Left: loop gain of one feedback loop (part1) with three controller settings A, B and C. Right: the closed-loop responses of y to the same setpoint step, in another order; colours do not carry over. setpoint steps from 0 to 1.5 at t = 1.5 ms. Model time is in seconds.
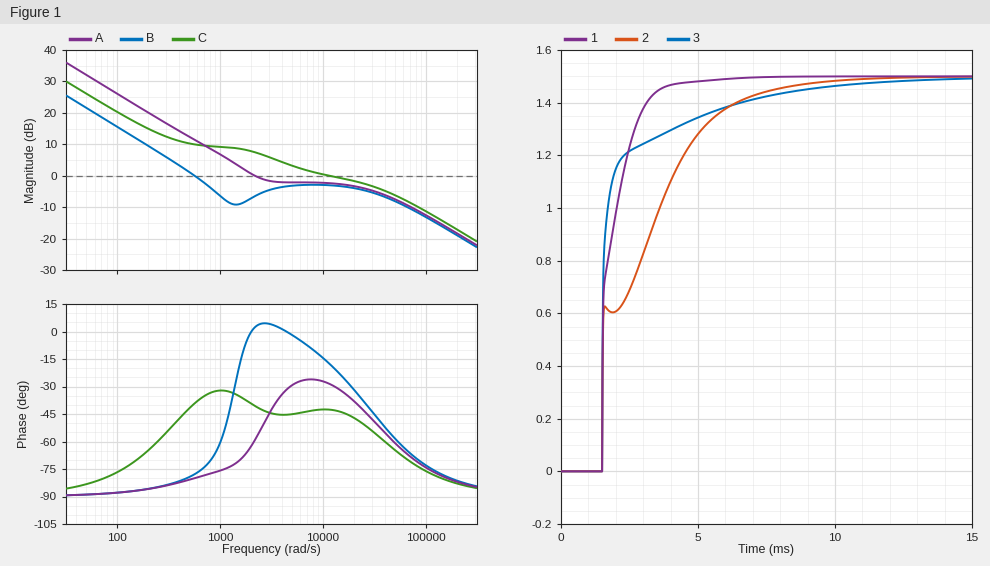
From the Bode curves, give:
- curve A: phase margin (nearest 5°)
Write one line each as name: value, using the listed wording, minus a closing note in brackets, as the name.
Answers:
curve A: phase margin: 120°
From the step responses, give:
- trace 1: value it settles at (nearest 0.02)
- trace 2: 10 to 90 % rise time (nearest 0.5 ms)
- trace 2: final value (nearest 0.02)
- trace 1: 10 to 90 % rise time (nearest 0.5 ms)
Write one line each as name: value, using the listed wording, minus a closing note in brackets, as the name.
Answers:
trace 1: value it settles at: 1.50
trace 2: 10 to 90 % rise time: 4.0 ms
trace 2: final value: 1.50
trace 1: 10 to 90 % rise time: 1.5 ms
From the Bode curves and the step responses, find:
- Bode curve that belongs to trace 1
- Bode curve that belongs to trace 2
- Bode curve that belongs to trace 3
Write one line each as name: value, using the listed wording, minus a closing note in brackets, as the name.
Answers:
Bode curve that belongs to trace 1: A
Bode curve that belongs to trace 2: B
Bode curve that belongs to trace 3: C
